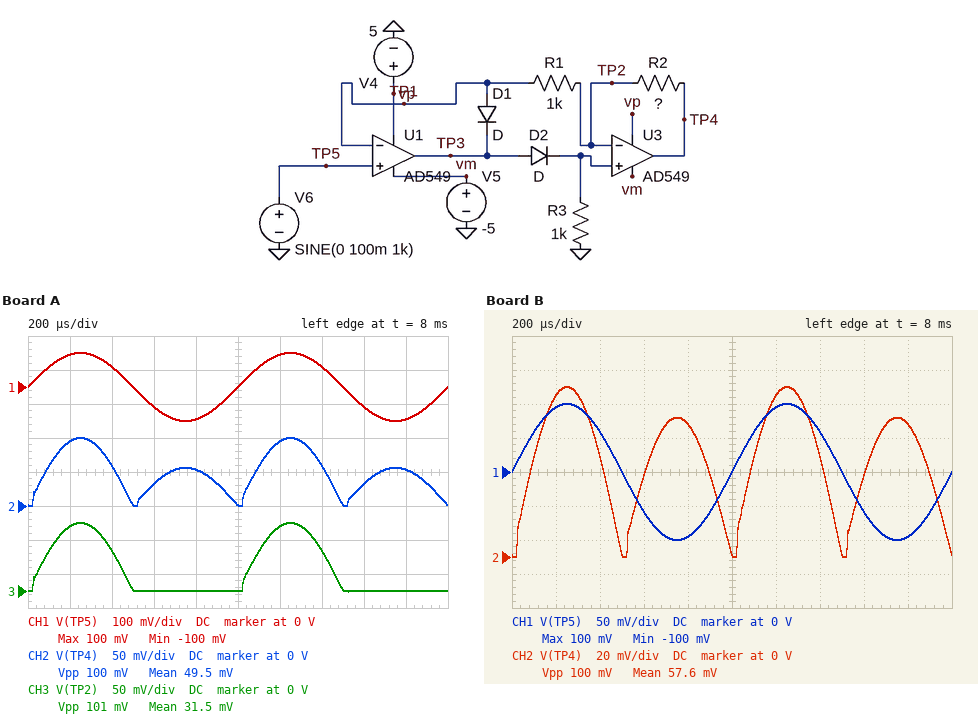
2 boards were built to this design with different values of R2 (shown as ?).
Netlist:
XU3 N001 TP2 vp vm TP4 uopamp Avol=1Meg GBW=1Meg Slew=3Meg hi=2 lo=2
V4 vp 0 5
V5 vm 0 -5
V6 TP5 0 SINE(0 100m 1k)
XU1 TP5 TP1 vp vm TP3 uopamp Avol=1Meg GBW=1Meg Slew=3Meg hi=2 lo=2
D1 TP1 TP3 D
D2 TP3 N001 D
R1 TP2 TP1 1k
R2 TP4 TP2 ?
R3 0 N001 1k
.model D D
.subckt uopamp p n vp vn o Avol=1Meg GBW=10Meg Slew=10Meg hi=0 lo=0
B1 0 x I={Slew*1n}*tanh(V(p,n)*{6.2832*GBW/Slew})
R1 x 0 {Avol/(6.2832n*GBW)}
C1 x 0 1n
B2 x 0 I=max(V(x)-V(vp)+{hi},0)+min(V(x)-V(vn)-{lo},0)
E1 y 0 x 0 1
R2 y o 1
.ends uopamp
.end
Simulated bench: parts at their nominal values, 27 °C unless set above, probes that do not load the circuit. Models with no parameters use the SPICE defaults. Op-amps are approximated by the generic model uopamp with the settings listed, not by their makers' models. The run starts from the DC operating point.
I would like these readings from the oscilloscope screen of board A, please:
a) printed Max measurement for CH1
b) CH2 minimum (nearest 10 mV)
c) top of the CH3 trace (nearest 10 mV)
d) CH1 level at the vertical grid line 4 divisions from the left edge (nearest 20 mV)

100 mV
0 V
100 mV
-100 mV
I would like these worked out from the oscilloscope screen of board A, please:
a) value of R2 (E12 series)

560 Ω
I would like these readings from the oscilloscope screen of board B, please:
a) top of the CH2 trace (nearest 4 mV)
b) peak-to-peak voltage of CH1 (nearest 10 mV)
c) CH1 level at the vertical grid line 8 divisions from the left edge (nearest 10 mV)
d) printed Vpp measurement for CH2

100 mV
200 mV
-60 mV
100 mV
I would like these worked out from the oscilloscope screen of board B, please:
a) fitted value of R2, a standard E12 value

820 Ω
